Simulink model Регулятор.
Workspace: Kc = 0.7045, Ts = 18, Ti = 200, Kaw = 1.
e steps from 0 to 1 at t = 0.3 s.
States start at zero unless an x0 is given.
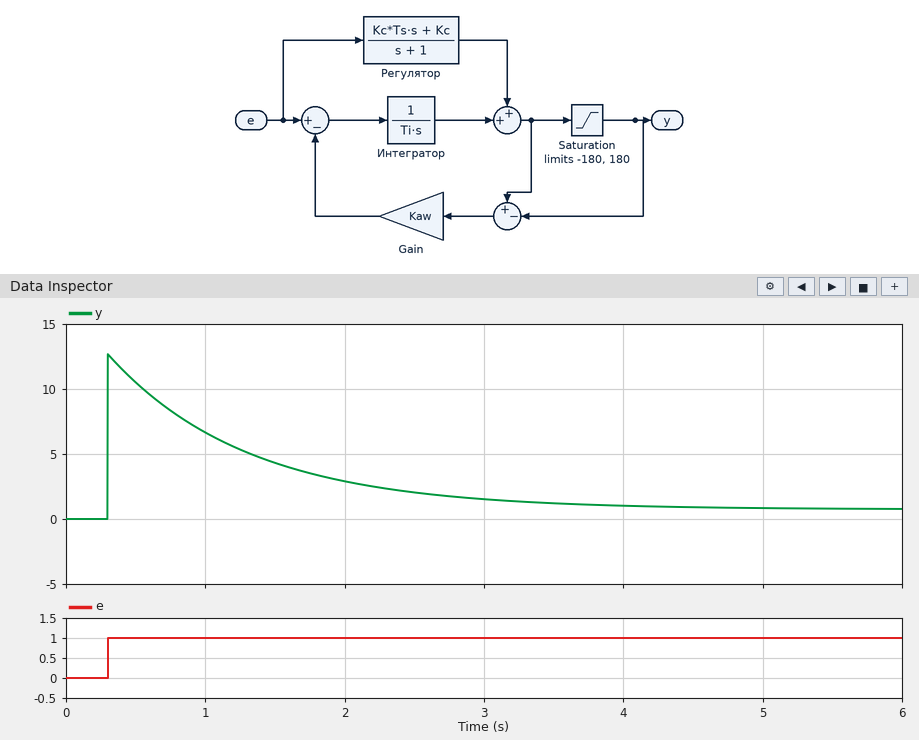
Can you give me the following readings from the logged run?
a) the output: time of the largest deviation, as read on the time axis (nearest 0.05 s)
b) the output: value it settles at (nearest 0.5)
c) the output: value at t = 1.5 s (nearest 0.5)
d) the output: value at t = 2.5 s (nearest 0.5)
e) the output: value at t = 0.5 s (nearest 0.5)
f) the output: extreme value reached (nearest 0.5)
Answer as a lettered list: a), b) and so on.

a) 0.30 s
b) 1.0
c) 4.5
d) 2.0
e) 10.5
f) 12.5
